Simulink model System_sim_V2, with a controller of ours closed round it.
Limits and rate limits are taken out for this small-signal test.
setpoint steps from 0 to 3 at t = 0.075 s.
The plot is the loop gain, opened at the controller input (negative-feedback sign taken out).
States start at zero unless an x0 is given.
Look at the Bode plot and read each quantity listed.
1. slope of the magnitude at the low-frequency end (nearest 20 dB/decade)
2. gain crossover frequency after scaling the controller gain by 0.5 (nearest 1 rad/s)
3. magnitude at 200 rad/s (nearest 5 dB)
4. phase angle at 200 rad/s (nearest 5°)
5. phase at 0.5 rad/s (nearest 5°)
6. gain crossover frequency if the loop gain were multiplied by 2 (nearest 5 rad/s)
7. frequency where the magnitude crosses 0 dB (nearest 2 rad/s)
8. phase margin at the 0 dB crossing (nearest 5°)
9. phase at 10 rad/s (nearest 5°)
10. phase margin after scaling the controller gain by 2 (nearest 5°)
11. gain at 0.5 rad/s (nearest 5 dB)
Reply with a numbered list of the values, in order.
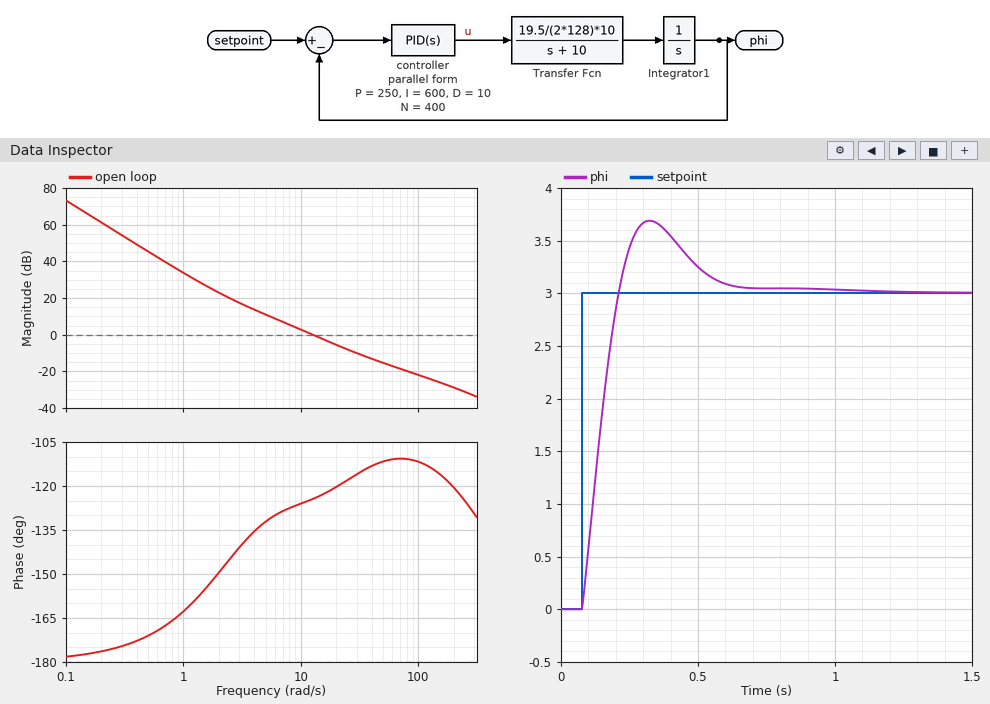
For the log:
1. -40 dB/decade
2. 8 rad/s
3. -30 dB
4. -120°
5. -170°
6. 20 rad/s
7. 12 rad/s
8. 55°
9. -125°
10. 60°
11. 45 dB
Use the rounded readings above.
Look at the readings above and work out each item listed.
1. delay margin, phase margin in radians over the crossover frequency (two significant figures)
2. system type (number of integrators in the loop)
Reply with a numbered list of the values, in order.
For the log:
1. 0.080 s
2. 2
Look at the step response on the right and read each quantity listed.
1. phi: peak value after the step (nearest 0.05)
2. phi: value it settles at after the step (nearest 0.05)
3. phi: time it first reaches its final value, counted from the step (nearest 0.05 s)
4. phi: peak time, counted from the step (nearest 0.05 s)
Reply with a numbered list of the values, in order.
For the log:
1. 3.70
2. 3.00
3. 0.15 s
4. 0.25 s
